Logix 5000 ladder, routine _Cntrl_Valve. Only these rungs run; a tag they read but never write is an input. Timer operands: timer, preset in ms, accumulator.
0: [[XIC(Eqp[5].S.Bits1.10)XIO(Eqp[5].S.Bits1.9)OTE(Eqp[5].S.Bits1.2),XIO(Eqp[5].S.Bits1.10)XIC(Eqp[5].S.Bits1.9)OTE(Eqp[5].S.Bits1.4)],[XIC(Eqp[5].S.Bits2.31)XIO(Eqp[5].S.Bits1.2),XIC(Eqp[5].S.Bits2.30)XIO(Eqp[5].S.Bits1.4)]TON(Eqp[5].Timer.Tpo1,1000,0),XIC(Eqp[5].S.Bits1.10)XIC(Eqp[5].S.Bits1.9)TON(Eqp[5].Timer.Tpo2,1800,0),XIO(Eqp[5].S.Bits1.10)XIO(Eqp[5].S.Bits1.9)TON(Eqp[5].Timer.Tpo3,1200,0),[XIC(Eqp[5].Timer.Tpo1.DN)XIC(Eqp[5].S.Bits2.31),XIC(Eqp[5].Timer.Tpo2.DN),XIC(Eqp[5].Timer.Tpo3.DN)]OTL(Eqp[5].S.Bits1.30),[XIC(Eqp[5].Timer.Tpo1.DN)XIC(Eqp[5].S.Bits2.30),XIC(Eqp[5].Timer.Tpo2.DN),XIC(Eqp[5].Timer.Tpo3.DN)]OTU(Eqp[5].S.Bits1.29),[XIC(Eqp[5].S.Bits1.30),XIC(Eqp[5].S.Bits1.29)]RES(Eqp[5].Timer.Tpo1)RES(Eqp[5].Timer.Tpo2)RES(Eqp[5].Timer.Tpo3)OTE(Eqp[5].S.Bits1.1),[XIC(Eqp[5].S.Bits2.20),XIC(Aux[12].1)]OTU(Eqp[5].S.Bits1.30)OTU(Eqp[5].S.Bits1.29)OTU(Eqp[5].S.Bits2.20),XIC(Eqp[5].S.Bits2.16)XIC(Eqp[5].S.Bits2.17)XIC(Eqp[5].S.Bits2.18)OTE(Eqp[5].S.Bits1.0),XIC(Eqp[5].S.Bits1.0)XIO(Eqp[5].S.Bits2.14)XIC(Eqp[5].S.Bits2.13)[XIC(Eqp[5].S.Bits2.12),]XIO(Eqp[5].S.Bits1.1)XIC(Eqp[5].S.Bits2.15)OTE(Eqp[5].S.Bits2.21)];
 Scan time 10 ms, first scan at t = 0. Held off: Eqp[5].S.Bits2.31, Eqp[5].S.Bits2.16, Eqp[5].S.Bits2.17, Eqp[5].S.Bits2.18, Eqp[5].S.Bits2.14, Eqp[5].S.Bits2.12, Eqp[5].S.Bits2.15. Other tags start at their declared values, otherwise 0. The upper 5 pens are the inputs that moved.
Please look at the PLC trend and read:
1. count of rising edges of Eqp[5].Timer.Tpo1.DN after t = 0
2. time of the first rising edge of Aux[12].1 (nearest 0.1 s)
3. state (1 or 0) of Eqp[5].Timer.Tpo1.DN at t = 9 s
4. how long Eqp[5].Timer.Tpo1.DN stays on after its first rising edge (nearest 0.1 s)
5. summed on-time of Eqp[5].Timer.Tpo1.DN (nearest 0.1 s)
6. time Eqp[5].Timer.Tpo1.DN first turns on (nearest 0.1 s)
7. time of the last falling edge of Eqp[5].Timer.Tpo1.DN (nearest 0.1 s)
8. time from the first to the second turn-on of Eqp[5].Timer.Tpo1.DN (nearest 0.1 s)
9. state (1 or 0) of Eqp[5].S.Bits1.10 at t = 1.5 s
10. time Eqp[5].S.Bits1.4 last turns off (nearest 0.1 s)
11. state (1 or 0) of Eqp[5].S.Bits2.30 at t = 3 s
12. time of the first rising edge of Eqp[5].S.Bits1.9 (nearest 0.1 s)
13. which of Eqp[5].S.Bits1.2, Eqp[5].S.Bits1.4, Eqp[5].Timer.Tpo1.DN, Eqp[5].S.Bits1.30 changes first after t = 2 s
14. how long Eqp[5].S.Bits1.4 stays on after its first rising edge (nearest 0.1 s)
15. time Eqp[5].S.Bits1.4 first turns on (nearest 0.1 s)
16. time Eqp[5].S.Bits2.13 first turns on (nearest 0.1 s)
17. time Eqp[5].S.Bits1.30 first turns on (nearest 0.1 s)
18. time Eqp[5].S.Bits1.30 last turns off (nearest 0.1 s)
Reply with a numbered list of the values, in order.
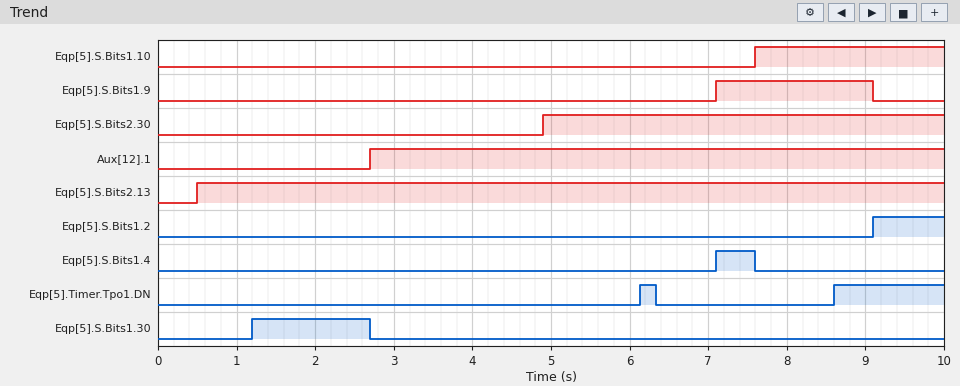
1. 2
2. 2.7 s
3. 1
4. 0.2 s
5. 1.6 s
6. 6.1 s
7. 6.3 s
8. 2.5 s
9. 0
10. 7.6 s
11. 0
12. 7.1 s
13. Eqp[5].S.Bits1.30
14. 0.5 s
15. 7.1 s
16. 0.5 s
17. 1.2 s
18. 2.7 s
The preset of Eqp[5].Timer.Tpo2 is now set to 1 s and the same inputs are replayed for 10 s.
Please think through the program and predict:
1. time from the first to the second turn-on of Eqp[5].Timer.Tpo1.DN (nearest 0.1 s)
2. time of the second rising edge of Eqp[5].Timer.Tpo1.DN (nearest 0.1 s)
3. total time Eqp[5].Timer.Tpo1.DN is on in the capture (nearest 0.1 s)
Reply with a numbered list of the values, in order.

1. 3.5 s
2. 9.6 s
3. 0.6 s
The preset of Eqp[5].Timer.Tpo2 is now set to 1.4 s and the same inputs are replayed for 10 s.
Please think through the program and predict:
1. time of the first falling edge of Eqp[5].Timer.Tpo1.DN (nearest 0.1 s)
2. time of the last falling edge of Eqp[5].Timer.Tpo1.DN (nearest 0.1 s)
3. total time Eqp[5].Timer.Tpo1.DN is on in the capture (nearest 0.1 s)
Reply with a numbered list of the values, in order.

1. 6.3 s
2. 9.0 s
3. 0.6 s
